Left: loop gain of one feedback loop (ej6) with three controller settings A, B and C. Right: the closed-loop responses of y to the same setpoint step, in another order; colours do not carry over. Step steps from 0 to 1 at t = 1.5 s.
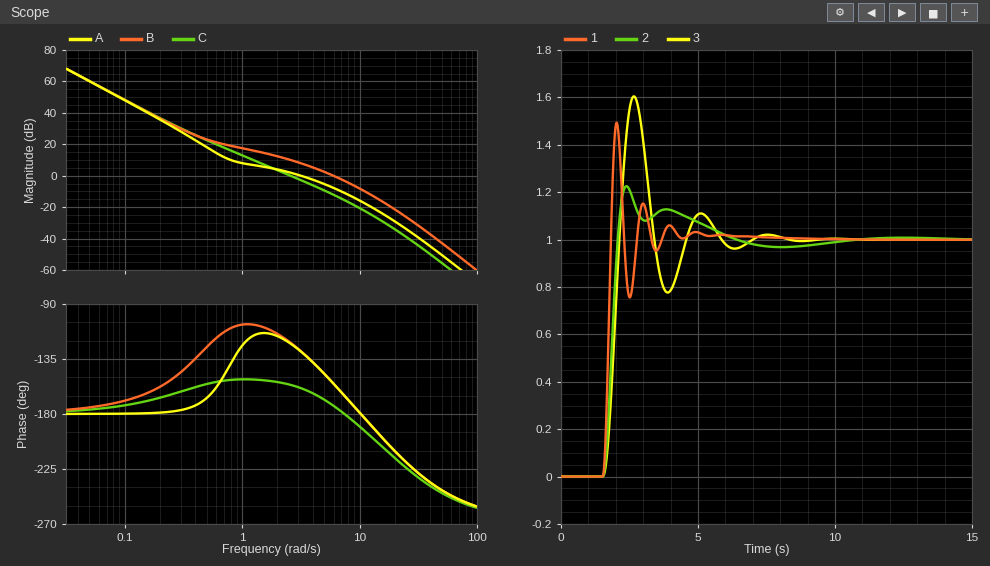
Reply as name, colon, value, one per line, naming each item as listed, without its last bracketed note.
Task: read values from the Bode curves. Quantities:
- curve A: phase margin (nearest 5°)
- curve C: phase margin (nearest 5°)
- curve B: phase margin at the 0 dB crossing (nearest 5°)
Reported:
curve A: phase margin: 50°
curve C: phase margin: 25°
curve B: phase margin at the 0 dB crossing: 25°
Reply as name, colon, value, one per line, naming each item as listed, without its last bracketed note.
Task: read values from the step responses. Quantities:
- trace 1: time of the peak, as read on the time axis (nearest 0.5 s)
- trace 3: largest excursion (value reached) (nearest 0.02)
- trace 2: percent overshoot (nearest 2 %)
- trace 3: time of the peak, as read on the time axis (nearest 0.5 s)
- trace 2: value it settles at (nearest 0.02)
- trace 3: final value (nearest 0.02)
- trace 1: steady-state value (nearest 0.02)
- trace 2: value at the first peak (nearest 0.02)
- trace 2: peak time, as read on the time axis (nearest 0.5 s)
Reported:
trace 1: time of the peak, as read on the time axis: 2.0 s
trace 3: largest excursion (value reached): 1.60
trace 2: percent overshoot: 22 %
trace 3: time of the peak, as read on the time axis: 2.5 s
trace 2: value it settles at: 1.00
trace 3: final value: 1.00
trace 1: steady-state value: 1.00
trace 2: value at the first peak: 1.22
trace 2: peak time, as read on the time axis: 2.5 s
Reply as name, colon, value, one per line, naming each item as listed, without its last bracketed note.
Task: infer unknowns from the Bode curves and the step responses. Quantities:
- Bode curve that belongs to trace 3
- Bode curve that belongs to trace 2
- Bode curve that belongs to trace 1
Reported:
Bode curve that belongs to trace 3: C
Bode curve that belongs to trace 2: A
Bode curve that belongs to trace 1: B
